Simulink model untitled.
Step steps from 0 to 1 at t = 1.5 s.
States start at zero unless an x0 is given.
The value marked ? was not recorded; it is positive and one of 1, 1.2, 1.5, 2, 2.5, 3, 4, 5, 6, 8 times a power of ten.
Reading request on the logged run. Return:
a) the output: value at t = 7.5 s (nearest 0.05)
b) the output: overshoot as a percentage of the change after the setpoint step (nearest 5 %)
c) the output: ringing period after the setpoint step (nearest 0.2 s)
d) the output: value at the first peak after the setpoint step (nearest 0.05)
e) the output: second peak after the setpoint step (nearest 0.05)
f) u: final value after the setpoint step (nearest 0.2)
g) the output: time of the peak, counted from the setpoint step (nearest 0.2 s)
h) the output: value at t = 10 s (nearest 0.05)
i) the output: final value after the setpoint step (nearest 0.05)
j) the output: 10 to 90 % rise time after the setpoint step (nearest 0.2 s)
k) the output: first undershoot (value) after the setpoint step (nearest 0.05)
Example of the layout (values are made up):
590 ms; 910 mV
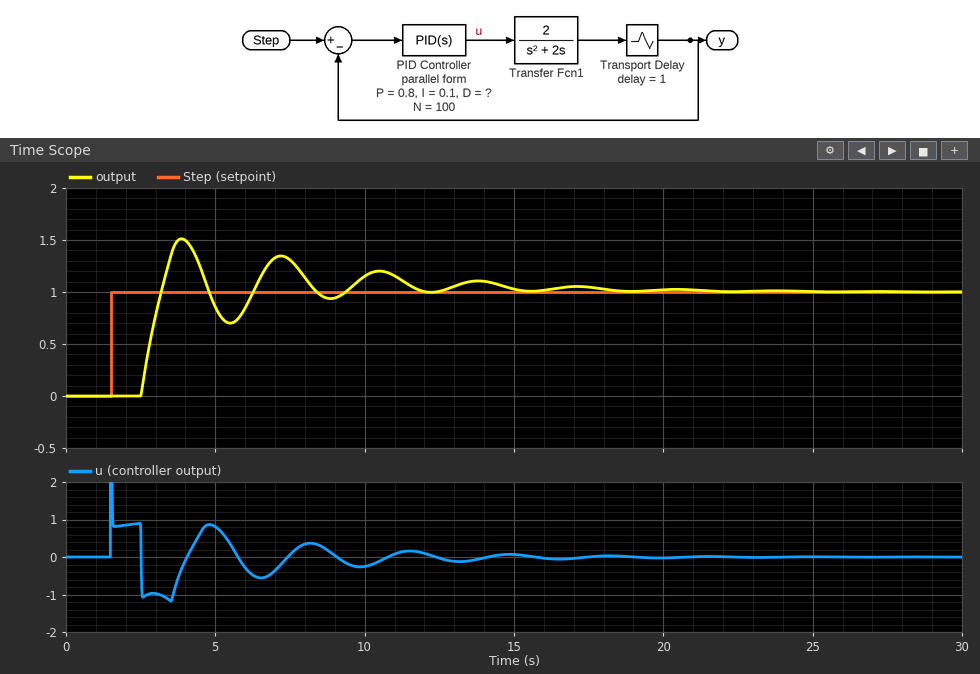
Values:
1.30; 50 %; 3.4 s; 1.50; 1.35; 0.0; 2.4 s; 1.15; 1.00; 0.6 s; 0.70
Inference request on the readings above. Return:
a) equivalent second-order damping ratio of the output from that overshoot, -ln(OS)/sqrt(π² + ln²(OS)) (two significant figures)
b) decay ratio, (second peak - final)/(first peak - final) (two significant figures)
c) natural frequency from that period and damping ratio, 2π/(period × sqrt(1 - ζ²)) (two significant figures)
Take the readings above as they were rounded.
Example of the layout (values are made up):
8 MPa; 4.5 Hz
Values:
0.22; 0.70; 1.9 rad/s
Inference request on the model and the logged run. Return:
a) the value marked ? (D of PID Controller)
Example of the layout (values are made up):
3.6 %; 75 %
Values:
1
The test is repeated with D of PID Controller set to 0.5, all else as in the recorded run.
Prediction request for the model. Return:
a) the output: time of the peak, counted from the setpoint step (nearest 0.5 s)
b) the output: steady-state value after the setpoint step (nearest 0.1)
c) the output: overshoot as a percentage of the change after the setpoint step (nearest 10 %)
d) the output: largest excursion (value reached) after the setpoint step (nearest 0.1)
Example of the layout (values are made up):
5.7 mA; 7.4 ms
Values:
3.0 s; 1.0; 40 %; 1.4
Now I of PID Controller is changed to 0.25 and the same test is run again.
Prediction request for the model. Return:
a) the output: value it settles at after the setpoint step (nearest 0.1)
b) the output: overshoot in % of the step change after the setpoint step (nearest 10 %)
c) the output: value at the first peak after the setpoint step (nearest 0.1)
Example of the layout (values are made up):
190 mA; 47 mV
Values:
1.0; 60 %; 1.6
